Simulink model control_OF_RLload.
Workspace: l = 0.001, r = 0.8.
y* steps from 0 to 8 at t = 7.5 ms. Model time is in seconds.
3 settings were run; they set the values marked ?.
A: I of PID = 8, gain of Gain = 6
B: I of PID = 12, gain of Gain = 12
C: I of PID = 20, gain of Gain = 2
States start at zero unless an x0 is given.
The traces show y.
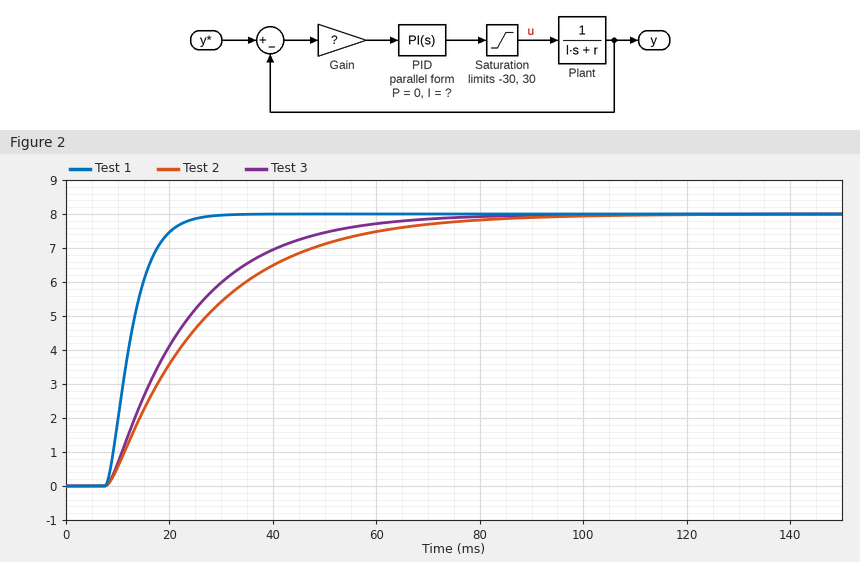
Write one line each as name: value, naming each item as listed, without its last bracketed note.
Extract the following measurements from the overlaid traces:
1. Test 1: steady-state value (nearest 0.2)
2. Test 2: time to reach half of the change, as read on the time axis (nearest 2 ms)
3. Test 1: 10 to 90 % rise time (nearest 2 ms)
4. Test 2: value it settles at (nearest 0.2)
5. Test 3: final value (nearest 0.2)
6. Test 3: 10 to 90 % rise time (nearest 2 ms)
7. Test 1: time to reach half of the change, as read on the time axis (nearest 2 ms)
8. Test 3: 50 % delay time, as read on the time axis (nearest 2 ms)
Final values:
Test 1: steady-state value: 8.0
Test 2: time to reach half of the change, as read on the time axis: 22 ms
Test 1: 10 to 90 % rise time: 10 ms
Test 2: value it settles at: 8.0
Test 3: final value: 8.0
Test 3: 10 to 90 % rise time: 34 ms
Test 1: time to reach half of the change, as read on the time axis: 12 ms
Test 3: 50 % delay time, as read on the time axis: 20 ms
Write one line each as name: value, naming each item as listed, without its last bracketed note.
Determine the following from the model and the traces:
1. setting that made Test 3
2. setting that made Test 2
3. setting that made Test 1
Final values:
setting that made Test 3: A
setting that made Test 2: C
setting that made Test 1: B
